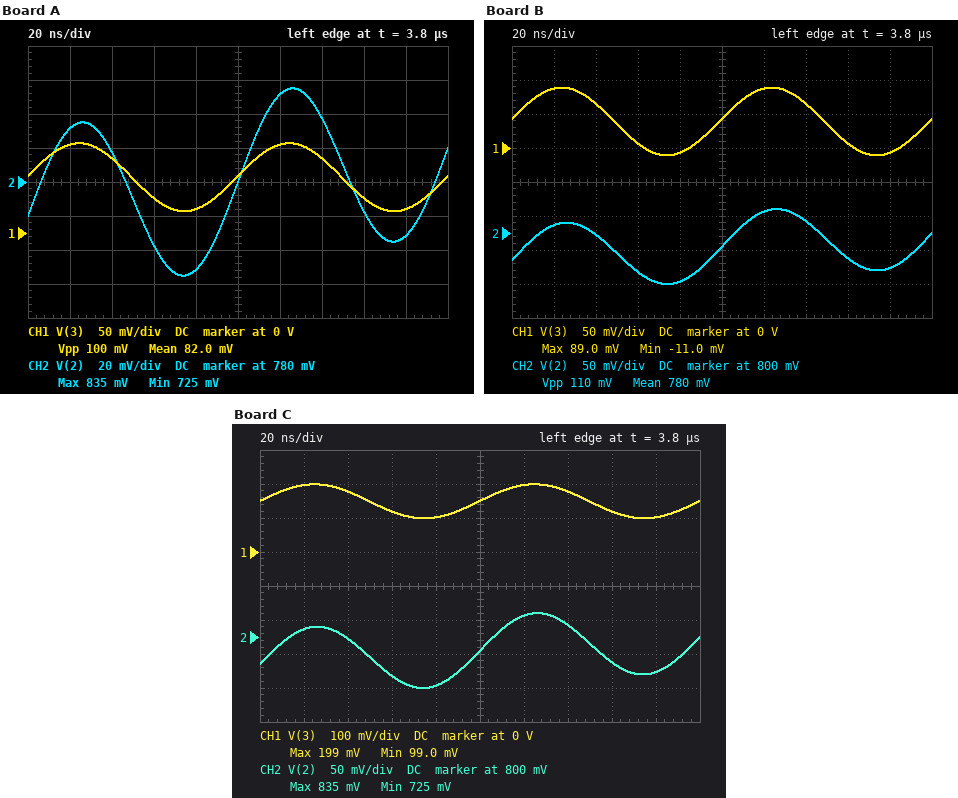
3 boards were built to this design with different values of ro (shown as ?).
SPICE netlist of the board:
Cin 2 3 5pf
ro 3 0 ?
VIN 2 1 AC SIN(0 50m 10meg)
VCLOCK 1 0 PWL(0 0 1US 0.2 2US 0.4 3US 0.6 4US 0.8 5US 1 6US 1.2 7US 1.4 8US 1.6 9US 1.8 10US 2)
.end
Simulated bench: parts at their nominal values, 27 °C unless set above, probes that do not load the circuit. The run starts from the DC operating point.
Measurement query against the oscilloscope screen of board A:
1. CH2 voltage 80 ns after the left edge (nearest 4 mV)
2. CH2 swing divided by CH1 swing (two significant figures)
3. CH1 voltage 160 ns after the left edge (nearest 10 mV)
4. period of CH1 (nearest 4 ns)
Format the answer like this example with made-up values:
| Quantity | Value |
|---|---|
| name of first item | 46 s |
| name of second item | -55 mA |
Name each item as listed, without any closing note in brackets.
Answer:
| Quantity | Value |
|---|---|
| CH2 voltage 80 ns after the left edge | 728 mV |
| CH2 swing divided by CH1 swing | 1.1 |
| CH1 voltage 160 ns after the left edge | 50 mV |
| period of CH1 | 100 ns |
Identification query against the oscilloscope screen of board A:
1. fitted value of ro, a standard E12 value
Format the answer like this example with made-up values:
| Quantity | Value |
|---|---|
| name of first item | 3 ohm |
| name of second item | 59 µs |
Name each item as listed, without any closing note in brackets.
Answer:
| Quantity | Value |
|---|---|
| fitted value of ro, a standard E12 value | 82 kΩ |
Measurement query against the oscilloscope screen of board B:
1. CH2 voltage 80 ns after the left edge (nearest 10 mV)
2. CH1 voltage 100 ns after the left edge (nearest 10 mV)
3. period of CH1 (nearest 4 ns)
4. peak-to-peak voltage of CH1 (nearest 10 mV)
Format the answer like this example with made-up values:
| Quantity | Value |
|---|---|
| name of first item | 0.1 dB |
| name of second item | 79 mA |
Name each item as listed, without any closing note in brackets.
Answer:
| Quantity | Value |
|---|---|
| CH2 voltage 80 ns after the left edge | 730 mV |
| CH1 voltage 100 ns after the left edge | 40 mV |
| period of CH1 | 100 ns |
| peak-to-peak voltage of CH1 | 100 mV |
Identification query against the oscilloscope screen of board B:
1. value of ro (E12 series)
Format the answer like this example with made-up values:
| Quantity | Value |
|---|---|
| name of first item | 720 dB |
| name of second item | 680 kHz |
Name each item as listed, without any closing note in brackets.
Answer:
| Quantity | Value |
|---|---|
| value of ro | 39 kΩ |
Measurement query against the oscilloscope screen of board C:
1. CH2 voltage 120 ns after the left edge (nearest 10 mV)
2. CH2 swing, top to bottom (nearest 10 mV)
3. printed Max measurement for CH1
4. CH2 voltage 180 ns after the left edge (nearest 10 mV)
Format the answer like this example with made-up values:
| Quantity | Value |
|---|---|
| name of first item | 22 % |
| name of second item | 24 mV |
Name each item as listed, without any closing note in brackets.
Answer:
| Quantity | Value |
|---|---|
| CH2 voltage 120 ns after the left edge | 830 mV |
| CH2 swing, top to bottom | 110 mV |
| printed Max measurement for CH1 | 199 mV |
| CH2 voltage 180 ns after the left edge | 750 mV |
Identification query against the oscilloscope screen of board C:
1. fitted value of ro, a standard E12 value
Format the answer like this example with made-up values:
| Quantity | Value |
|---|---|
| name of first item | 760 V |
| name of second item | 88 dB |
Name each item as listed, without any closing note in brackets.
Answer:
| Quantity | Value |
|---|---|
| fitted value of ro, a standard E12 value | 150 kΩ |
